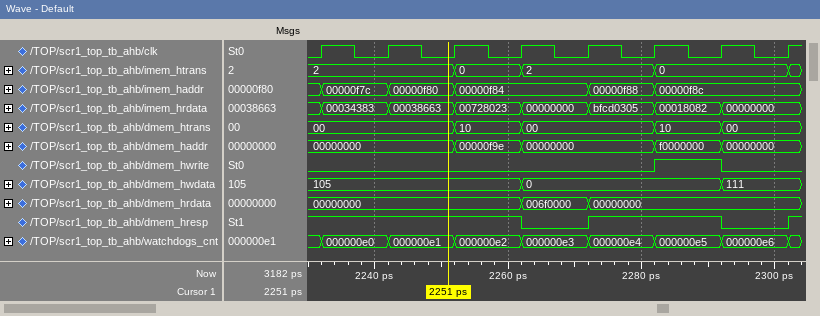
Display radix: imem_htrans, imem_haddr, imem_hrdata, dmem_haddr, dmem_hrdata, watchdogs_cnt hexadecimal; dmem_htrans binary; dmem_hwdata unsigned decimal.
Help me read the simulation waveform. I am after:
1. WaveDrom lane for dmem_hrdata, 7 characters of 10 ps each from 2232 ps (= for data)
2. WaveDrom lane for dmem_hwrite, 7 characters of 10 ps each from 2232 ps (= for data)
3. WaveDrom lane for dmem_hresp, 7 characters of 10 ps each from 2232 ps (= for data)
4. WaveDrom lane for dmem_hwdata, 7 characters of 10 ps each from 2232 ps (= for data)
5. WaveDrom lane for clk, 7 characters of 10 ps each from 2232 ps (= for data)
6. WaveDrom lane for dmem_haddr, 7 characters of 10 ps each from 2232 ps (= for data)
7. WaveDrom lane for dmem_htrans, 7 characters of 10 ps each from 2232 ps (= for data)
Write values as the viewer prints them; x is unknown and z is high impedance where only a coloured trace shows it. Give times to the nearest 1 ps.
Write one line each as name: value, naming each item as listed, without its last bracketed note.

WaveDrom lane for dmem_hrdata, 7 characters of 10 ps each from 2232 ps: {name: 'dmem_hrdata', wave: '=..==..', data: '00000000 006f0000 00000000'}
WaveDrom lane for dmem_hwrite, 7 characters of 10 ps each from 2232 ps: {name: 'dmem_hwrite', wave: '0....10'}
WaveDrom lane for dmem_hresp, 7 characters of 10 ps each from 2232 ps: {name: 'dmem_hresp', wave: '1..01.0'}
WaveDrom lane for dmem_hwdata, 7 characters of 10 ps each from 2232 ps: {name: 'dmem_hwdata', wave: '=..=..=', data: '105 0 111'}
WaveDrom lane for clk, 7 characters of 10 ps each from 2232 ps: {name: 'clk', wave: 'p......'}
WaveDrom lane for dmem_haddr, 7 characters of 10 ps each from 2232 ps: {name: 'dmem_haddr', wave: '=.==.==', data: '00000000 00000f9e 00000000 f0000000 00000000'}
WaveDrom lane for dmem_htrans, 7 characters of 10 ps each from 2232 ps: {name: 'dmem_htrans', wave: '=.==.==', data: '00 10 00 10 00'}
